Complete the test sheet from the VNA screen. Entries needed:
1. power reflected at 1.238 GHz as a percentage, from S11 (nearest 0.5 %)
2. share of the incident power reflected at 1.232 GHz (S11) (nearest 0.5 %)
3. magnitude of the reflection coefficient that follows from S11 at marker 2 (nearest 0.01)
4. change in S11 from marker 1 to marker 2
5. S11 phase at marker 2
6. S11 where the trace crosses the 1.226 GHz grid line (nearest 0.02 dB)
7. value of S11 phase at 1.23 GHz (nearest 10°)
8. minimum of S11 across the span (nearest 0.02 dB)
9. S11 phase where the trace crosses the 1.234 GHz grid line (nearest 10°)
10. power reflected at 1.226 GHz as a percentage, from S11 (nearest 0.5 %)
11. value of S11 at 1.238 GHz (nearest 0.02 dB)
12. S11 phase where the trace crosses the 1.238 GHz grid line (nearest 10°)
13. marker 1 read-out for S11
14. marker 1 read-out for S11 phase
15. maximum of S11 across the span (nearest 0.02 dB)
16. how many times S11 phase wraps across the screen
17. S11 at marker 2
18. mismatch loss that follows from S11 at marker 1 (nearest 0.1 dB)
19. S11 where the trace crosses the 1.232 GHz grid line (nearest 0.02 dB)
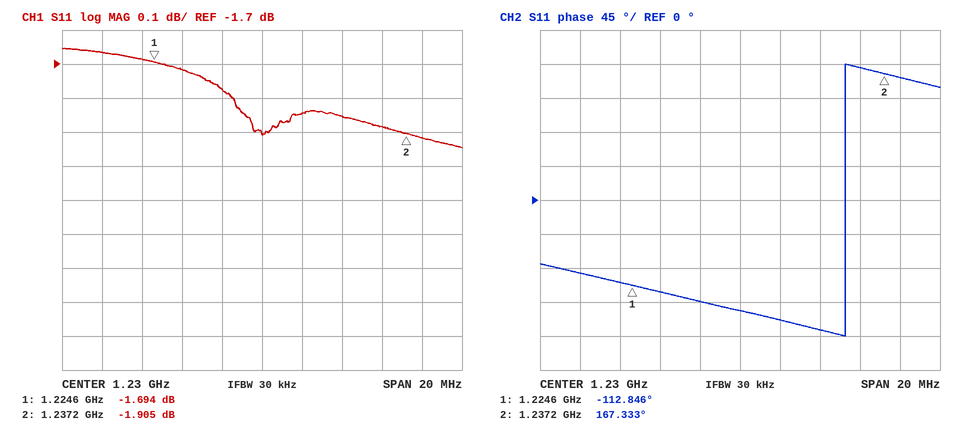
64.5 %
65.5 %
0.80
-0.211 dB
167.333°
-1.72 dB
-150°
-1.94 dB
-170°
67.5 %
-1.92 dB
160°
-1.694 dB
-112.846°
-1.66 dB
1
-1.905 dB
4.9 dB
-1.84 dB
